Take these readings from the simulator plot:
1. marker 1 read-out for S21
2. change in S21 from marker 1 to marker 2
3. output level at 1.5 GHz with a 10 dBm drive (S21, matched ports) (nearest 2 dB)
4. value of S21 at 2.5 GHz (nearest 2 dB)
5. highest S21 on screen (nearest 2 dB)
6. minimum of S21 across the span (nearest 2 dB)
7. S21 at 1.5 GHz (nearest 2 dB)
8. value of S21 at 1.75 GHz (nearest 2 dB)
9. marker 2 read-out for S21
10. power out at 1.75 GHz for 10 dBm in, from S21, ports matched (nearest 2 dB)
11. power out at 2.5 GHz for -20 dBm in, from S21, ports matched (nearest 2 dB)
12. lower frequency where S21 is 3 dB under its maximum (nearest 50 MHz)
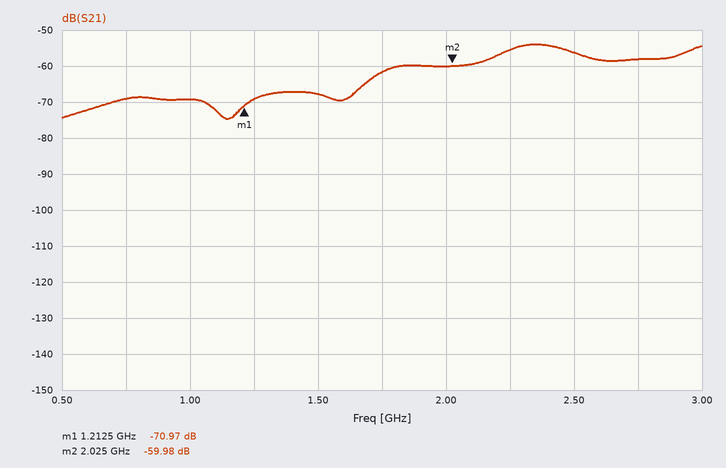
-70.97 dB
10.99 dB
-58 dBm
-56 dB
-54 dB
-74 dB
-68 dB
-62 dB
-59.98 dB
-52 dBm
-76 dBm
2.20 GHz
